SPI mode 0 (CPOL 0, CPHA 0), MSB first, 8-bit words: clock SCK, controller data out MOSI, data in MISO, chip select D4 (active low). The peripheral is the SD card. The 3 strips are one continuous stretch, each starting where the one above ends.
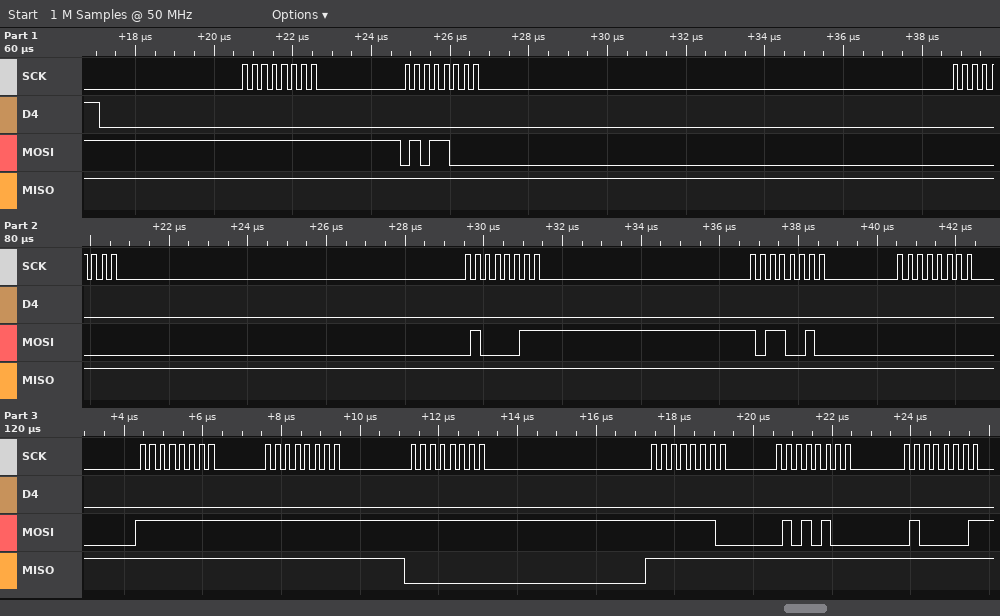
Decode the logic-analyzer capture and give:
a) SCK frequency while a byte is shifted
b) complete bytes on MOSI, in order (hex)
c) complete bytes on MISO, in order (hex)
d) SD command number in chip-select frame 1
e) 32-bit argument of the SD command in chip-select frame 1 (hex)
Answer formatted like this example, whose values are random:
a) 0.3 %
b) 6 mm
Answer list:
a) 4 MHz
b) 0xFF 0x58 0x00 0x43 0xB2 0x00 0xFF 0xFF 0xFF 0xFE 0x54 0x41
c) 0xFF 0xFF 0xFF 0xFF 0xFF 0xFF 0xFF 0xFF 0x00 0xFF 0xFF 0xFF
d) CMD24
e) 0x0043B200
